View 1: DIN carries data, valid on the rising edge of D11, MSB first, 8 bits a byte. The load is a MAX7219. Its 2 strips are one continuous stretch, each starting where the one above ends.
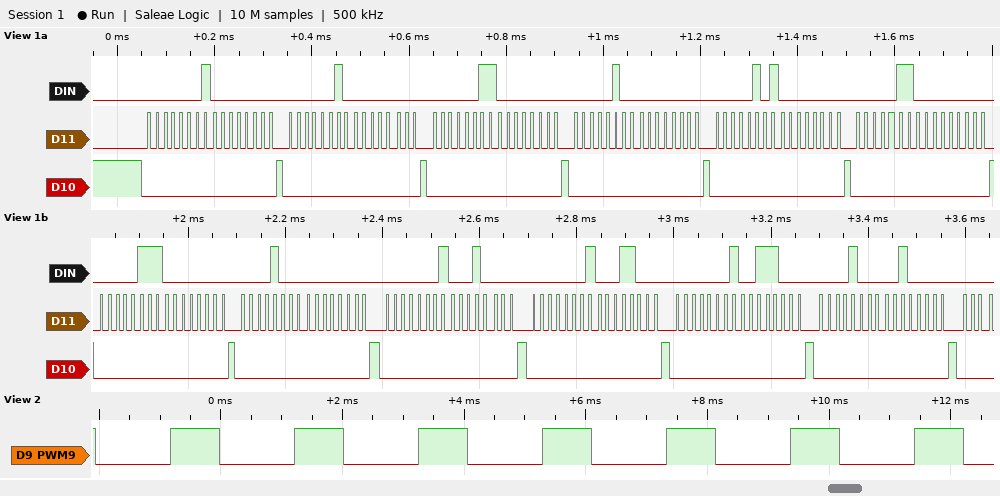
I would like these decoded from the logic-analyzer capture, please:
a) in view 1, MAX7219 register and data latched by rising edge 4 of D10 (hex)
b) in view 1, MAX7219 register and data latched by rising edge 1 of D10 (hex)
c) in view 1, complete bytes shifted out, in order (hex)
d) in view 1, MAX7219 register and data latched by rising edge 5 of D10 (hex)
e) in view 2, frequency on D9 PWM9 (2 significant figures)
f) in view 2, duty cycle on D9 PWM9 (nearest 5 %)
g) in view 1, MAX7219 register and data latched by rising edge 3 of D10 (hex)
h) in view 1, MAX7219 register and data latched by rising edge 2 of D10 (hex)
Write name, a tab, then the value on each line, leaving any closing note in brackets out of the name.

in view 1, MAX7219 register and data latched by rising edge 4 of D10	register 0x4, data 0x00
in view 1, MAX7219 register and data latched by rising edge 1 of D10	register 0x1, data 0x00
in view 1, complete bytes shifted out, in order	01 00 02 00 03 00 04 00 05 00 06 00 07 00 08 00 01 10 01 18 01 38 08 20
in view 1, MAX7219 register and data latched by rising edge 5 of D10	register 0x5, data 0x00
in view 2, frequency on D9 PWM9	490 Hz
in view 2, duty cycle on D9 PWM9	40 %
in view 1, MAX7219 register and data latched by rising edge 3 of D10	register 0x3, data 0x00
in view 1, MAX7219 register and data latched by rising edge 2 of D10	register 0x2, data 0x00
